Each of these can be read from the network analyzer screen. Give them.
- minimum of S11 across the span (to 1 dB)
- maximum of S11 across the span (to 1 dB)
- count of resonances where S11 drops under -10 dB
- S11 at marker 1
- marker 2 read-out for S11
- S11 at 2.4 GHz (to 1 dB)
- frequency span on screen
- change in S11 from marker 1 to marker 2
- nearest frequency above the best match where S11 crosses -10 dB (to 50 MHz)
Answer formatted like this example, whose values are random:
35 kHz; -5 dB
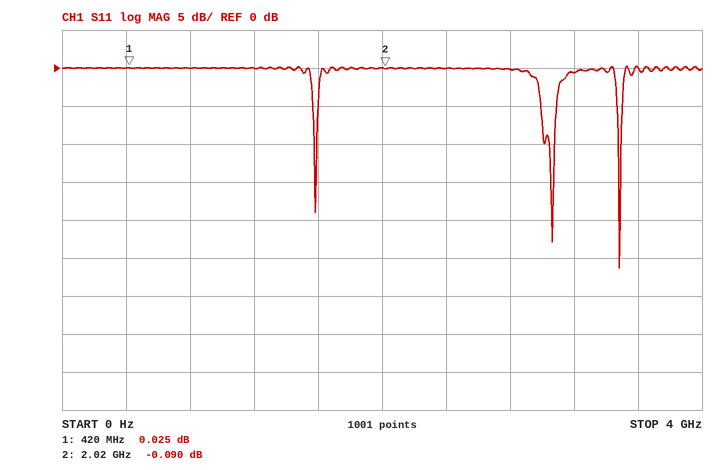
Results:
-26 dB; 0 dB; 3; 0.025 dB; -0.090 dB; 0 dB; 4 GHz; -0.115 dB; 3.50 GHz
